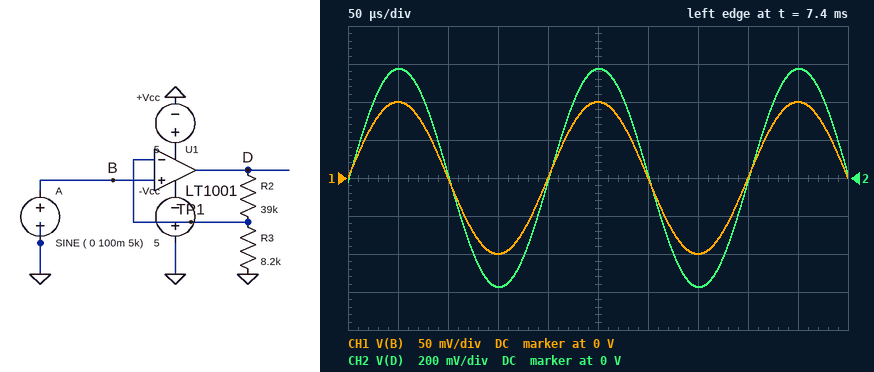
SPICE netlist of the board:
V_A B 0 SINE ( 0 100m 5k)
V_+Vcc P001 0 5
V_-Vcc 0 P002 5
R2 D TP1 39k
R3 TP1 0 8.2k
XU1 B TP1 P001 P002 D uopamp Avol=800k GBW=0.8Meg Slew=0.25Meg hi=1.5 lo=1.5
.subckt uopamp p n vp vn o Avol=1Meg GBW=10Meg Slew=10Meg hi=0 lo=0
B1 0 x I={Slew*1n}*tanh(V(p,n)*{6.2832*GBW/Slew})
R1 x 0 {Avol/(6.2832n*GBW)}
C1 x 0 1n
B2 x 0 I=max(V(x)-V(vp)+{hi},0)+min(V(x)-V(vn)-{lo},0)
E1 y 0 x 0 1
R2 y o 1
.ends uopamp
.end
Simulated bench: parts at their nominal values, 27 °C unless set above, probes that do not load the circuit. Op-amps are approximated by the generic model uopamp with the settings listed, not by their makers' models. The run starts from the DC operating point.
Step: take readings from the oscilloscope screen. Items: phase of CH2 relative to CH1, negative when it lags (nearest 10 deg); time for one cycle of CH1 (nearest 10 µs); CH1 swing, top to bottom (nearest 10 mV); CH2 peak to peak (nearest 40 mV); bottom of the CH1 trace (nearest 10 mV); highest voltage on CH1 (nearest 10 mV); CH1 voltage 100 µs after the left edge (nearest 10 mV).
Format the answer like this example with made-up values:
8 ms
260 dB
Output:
0 deg
200 µs
200 mV
1.16 V
-100 mV
100 mV
0 V
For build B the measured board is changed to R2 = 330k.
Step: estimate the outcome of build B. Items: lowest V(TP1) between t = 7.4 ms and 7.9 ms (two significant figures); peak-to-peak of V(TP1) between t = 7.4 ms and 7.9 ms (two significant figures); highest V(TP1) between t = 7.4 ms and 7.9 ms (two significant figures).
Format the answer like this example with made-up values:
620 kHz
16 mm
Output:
-85 mV
170 mV
85 mV
